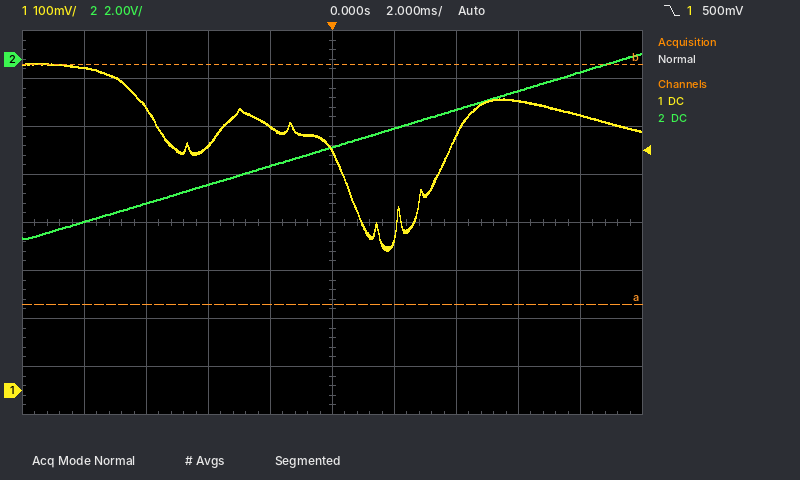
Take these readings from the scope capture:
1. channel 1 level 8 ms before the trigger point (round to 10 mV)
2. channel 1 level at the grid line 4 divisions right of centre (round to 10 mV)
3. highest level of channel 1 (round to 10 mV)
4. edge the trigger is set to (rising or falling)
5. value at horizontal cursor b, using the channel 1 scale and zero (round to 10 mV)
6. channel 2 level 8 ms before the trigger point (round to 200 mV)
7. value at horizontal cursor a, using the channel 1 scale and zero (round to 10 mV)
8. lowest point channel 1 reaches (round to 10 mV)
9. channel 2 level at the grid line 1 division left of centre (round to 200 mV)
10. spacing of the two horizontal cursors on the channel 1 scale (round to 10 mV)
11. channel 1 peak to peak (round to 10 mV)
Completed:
670 mV
570 mV
680 mV
falling
680 mV
-6.8 V
180 mV
290 mV
-4.4 V
500 mV
390 mV
